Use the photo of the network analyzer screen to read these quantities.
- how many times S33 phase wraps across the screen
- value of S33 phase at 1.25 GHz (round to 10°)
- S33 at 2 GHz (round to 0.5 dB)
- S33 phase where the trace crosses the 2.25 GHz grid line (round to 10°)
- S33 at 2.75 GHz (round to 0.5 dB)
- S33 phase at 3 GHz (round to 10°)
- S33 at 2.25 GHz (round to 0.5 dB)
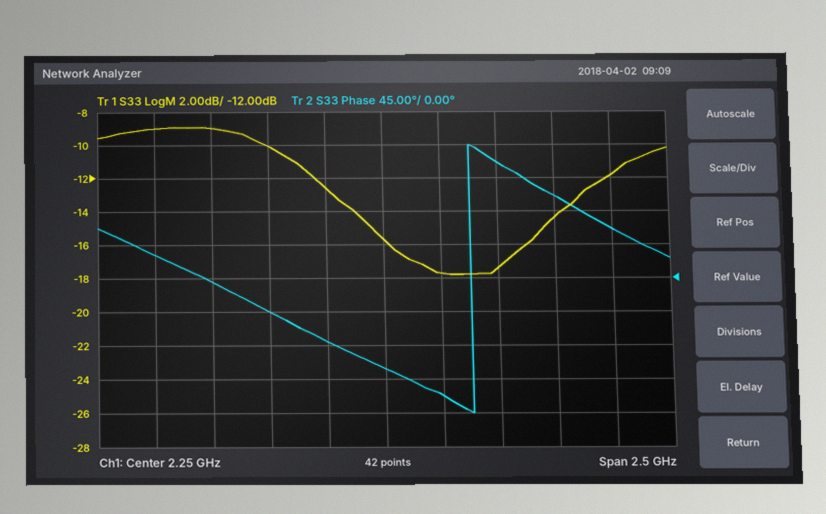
1
30°
-12.5 dB
-120°
-17.5 dB
110°
-15.5 dB
